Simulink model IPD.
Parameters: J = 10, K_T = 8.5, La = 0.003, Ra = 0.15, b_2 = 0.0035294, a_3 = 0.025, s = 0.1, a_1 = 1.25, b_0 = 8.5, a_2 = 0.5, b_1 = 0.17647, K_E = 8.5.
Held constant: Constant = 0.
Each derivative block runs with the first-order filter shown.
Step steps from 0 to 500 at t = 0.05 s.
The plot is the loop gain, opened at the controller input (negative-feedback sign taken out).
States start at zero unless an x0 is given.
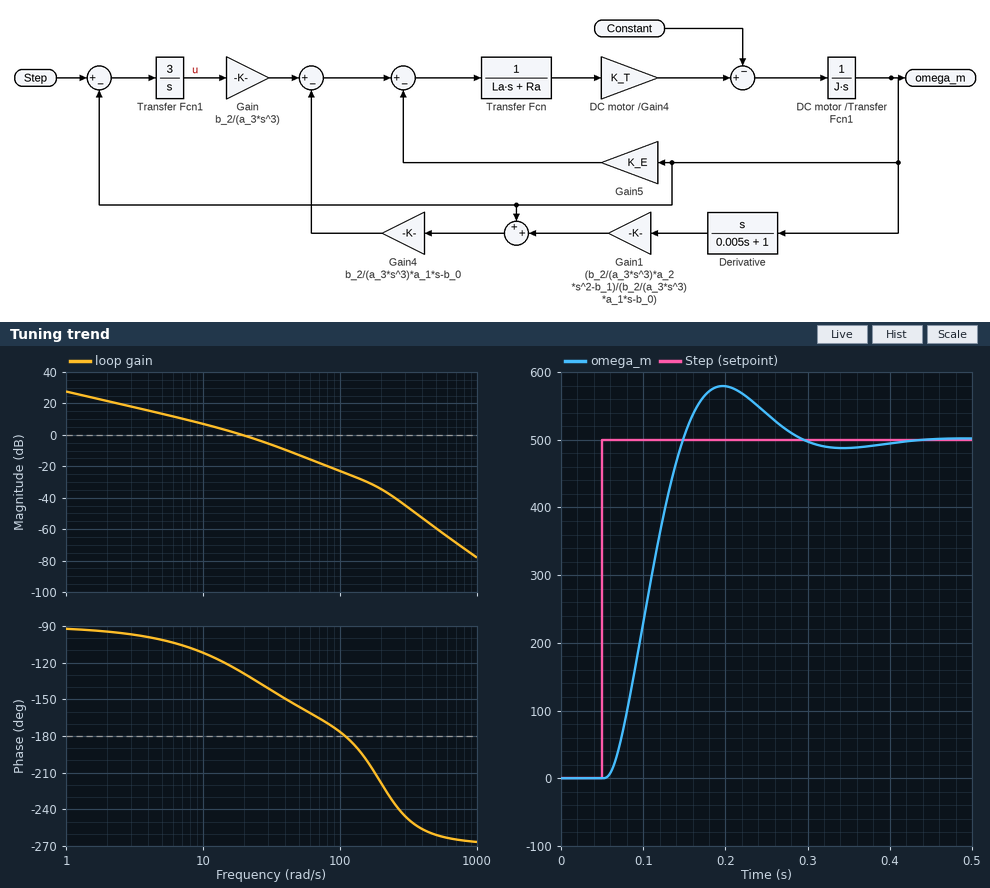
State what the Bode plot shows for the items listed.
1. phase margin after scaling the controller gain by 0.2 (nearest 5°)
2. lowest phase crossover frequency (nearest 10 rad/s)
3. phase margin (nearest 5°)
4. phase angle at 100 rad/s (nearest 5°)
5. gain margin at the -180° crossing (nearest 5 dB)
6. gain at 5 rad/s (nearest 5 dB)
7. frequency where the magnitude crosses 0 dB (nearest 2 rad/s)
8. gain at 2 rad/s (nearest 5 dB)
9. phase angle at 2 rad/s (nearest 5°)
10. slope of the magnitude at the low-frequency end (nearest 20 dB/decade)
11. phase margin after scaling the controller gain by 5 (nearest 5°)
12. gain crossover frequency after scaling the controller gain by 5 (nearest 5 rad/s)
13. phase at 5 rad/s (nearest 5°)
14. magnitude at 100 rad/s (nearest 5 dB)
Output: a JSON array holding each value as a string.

["80°", "110 rad/s", "50°", "-175°", "25 dB", "15 dB", "20 rad/s", "20 dB", "-95°", "-20 dB/decade", "20°", "55 rad/s", "-100°", "-25 dB"]
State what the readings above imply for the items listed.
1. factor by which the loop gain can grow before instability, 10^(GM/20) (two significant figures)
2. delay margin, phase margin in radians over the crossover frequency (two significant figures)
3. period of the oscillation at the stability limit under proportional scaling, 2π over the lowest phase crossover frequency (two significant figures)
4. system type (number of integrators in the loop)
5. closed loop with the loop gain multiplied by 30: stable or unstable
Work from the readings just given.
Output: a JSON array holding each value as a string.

["18", "0.044 s", "0.057 s", "1", "unstable"]
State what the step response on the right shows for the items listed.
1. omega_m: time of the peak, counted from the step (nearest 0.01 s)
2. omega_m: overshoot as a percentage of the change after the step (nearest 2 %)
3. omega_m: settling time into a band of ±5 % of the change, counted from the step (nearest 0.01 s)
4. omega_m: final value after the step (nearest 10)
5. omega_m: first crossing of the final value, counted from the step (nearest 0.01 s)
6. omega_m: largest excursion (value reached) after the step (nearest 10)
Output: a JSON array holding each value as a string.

["0.15 s", "16 %", "0.21 s", "500", "0.10 s", "580"]
